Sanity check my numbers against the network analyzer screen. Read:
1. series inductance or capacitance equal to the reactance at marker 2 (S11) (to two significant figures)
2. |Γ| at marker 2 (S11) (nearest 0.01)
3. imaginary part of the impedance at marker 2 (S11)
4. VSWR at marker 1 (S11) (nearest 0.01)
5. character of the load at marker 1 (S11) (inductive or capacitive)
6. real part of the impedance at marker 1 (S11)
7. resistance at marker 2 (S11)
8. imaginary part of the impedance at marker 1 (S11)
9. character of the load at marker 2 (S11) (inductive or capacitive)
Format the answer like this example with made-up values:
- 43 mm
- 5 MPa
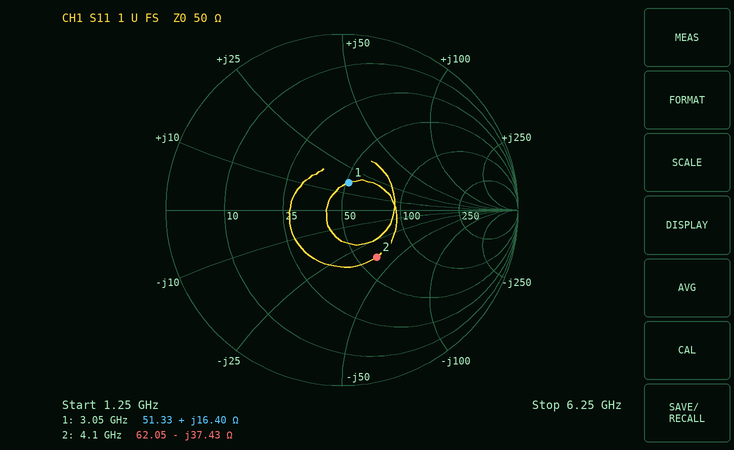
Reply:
- 1.0 pF
- 0.33
- -37.43 Ω
- 1.38
- inductive
- 51.33 Ω
- 62.05 Ω
- +16.40 Ω
- capacitive
